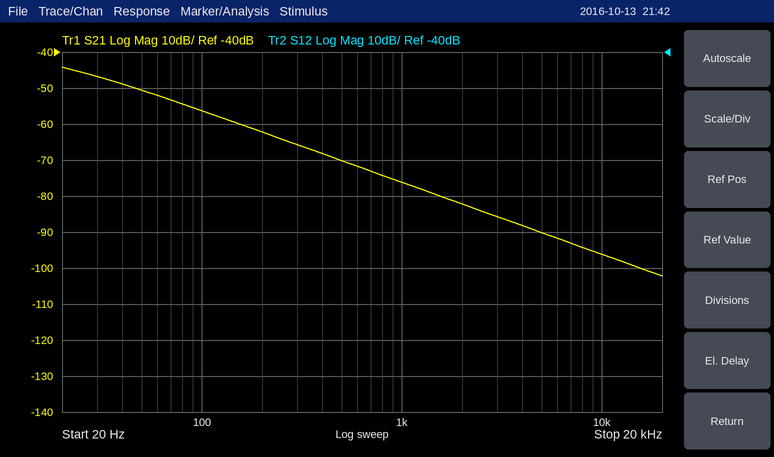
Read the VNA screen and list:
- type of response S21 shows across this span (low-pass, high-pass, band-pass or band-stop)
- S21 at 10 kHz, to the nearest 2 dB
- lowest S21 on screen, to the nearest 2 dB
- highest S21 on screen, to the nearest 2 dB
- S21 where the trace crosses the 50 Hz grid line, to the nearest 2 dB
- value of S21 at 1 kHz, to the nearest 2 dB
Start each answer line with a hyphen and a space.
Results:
- low-pass
- -96 dB
- -102 dB
- -44 dB
- -50 dB
- -76 dB
